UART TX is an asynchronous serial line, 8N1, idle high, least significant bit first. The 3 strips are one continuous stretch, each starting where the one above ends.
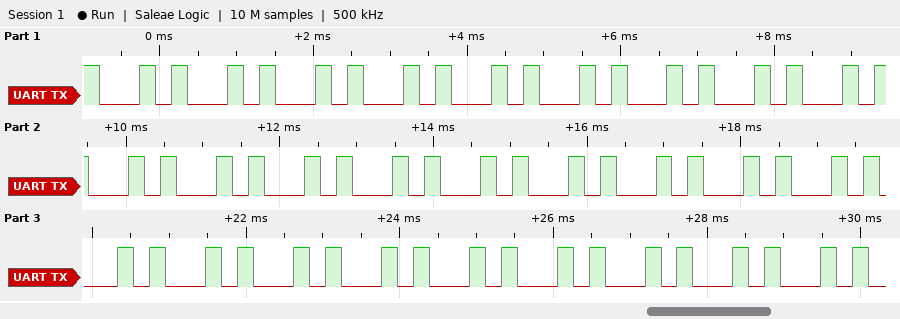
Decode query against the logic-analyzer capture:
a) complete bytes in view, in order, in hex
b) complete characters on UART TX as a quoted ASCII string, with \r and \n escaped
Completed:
30 30 30 30 30 30 30 30 30 30 30 30 30 30 30 30 30 30 30 30 30 30 30 30 30 30 30
"000000000000000000000000000"
